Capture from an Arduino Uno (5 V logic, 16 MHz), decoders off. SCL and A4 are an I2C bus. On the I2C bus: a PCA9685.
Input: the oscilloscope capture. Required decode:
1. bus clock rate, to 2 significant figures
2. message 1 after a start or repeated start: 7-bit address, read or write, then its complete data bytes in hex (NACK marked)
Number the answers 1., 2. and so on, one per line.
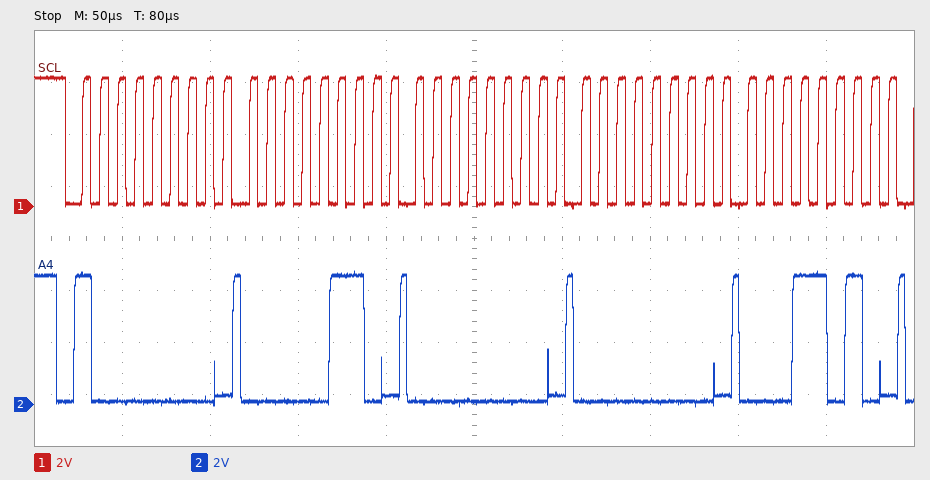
1. 100 kHz
2. 0x40 write: 06 00 00 1A
